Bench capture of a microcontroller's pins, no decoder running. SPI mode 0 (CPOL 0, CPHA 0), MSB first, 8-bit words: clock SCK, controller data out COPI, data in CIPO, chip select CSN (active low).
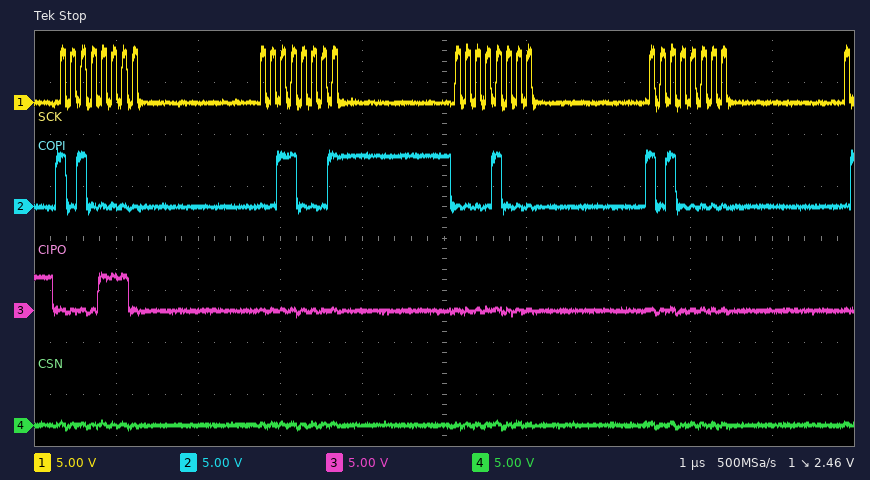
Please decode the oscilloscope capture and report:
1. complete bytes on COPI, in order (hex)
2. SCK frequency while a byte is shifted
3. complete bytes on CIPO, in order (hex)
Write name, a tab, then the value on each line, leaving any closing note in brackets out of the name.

complete bytes on COPI, in order	A0 31 08 A0
SCK frequency while a byte is shifted	8 MHz
complete bytes on CIPO, in order	0E 00 00 00
